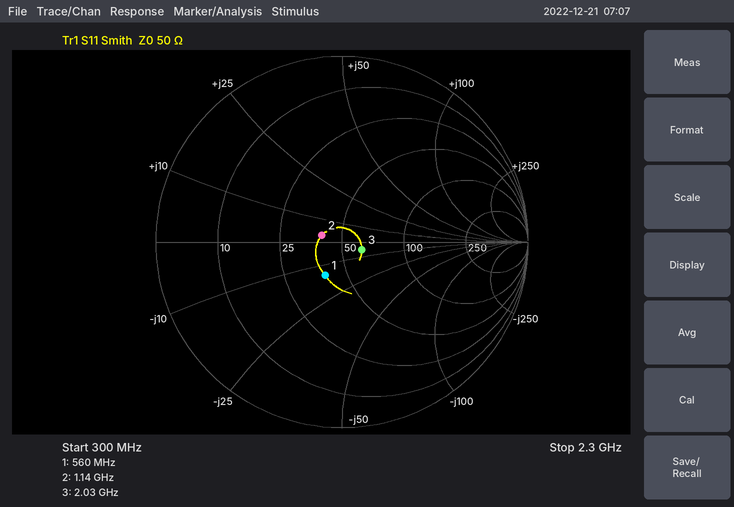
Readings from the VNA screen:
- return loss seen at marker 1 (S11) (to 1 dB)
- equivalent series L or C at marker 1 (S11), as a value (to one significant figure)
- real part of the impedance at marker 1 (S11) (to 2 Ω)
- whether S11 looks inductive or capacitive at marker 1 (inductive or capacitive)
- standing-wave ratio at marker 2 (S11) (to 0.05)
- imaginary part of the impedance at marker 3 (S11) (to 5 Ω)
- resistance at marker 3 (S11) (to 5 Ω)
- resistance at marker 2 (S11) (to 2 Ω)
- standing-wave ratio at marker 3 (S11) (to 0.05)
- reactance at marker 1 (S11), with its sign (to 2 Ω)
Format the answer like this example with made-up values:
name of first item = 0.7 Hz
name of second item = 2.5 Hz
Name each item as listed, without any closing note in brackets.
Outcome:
return loss seen at marker 1 (S11) = 14 dB
equivalent series L or C at marker 1 (S11), as a value = 20 pF
real part of the impedance at marker 1 (S11) = 40 Ω
whether S11 looks inductive or capacitive at marker 1 = capacitive
standing-wave ratio at marker 2 (S11) = 1.25
imaginary part of the impedance at marker 3 (S11) = -5 Ω
resistance at marker 3 (S11) = 60 Ω
resistance at marker 2 (S11) = 40 Ω
standing-wave ratio at marker 3 (S11) = 1.25
reactance at marker 1 (S11), with its sign = -14 Ω
